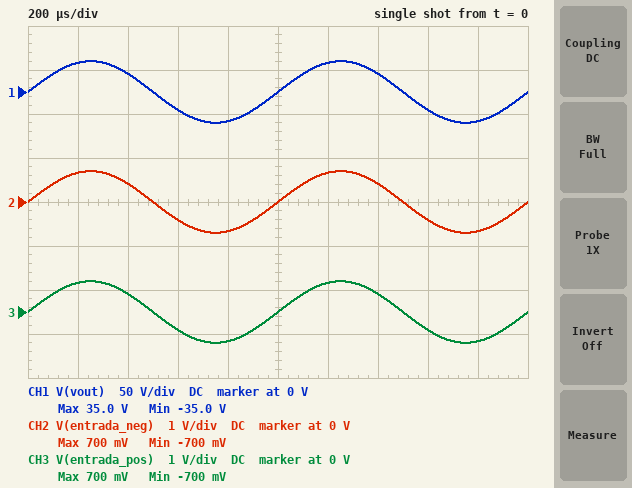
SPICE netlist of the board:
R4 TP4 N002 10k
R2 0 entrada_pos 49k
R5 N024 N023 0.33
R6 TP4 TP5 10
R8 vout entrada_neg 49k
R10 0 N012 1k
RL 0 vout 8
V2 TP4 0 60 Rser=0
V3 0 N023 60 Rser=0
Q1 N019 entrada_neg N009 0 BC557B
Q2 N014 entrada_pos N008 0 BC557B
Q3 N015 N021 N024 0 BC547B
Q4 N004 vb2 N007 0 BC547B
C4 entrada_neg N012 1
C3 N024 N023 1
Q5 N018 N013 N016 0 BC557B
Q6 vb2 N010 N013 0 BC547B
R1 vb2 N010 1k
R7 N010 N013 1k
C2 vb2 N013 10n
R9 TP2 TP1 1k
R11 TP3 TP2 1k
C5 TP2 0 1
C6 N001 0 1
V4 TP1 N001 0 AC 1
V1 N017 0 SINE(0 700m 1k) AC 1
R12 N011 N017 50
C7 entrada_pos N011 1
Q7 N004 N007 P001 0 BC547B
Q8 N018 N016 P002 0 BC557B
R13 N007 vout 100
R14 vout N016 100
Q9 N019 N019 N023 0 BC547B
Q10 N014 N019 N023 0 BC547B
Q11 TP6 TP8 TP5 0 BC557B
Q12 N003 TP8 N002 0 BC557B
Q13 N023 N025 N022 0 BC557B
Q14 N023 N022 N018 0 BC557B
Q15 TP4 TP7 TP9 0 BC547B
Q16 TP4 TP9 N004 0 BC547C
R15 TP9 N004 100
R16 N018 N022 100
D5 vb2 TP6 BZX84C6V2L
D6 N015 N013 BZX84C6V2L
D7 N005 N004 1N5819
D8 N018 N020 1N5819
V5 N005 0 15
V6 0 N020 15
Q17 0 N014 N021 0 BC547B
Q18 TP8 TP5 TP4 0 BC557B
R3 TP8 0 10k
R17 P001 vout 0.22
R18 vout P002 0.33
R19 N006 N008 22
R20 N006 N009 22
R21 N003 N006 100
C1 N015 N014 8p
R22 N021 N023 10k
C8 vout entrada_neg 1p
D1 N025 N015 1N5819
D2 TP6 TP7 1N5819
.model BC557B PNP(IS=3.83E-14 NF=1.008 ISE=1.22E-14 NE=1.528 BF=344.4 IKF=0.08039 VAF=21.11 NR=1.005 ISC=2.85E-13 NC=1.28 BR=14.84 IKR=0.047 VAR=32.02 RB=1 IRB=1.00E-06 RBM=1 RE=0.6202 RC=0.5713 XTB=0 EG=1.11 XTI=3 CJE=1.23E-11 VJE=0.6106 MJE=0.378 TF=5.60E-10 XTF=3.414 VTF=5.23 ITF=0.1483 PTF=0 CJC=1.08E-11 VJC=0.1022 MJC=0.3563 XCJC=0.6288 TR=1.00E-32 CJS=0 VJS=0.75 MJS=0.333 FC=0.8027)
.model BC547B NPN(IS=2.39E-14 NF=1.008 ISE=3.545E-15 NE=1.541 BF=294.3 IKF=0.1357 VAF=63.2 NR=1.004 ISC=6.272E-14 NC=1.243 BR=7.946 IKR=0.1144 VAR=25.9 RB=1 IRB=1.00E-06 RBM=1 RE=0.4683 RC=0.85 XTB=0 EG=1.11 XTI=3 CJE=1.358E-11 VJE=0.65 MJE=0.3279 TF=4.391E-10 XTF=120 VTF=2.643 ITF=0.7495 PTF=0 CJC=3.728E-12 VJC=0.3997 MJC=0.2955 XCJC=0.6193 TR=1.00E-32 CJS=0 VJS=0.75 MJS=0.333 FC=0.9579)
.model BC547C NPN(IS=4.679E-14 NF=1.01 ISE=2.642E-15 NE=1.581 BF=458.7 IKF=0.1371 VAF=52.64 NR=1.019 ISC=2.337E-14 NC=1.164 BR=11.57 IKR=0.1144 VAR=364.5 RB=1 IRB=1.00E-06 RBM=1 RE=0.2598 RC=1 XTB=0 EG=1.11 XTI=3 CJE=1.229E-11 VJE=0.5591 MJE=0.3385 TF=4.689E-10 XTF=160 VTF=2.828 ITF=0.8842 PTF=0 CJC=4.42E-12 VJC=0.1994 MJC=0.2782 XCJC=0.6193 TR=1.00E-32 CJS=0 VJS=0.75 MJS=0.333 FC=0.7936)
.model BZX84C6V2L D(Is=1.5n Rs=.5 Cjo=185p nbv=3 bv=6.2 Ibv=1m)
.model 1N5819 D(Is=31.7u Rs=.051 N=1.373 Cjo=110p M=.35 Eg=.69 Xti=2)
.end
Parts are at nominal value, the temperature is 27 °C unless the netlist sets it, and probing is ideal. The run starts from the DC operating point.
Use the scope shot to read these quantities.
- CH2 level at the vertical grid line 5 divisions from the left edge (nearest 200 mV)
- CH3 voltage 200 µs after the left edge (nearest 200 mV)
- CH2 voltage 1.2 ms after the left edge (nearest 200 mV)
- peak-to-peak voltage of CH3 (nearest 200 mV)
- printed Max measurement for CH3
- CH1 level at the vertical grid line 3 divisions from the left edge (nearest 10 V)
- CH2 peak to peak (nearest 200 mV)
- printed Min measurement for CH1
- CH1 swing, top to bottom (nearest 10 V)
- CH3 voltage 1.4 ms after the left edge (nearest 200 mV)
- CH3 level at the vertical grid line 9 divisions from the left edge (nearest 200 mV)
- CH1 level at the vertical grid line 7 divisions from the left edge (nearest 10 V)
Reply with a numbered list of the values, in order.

1. 0 V
2. 600 mV
3. 600 mV
4. 1.4 V
5. 700 mV
6. -20 V
7. 1.4 V
8. -35.0 V
9. 70 V
10. 400 mV
11. -600 mV
12. 20 V
